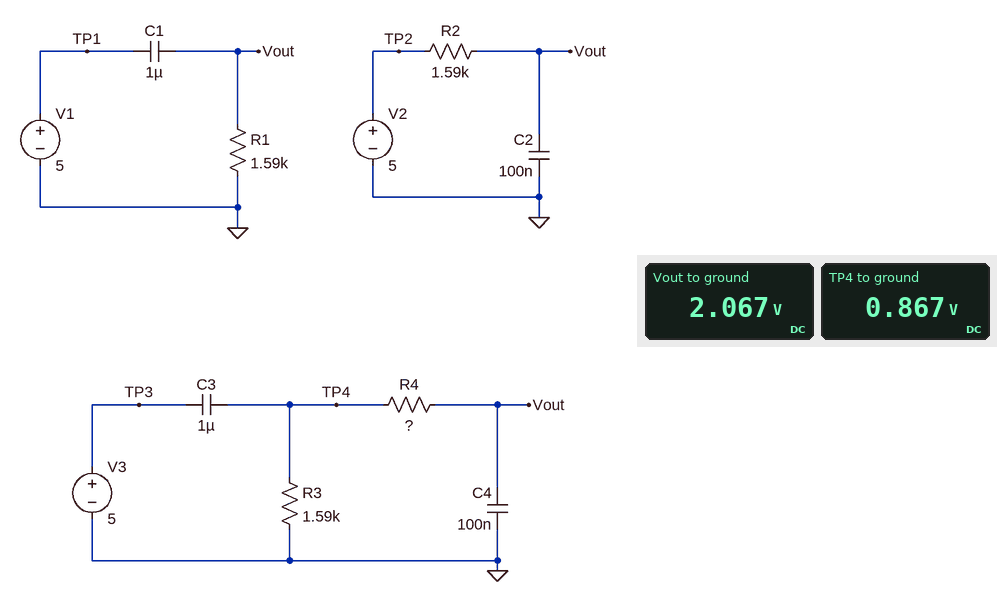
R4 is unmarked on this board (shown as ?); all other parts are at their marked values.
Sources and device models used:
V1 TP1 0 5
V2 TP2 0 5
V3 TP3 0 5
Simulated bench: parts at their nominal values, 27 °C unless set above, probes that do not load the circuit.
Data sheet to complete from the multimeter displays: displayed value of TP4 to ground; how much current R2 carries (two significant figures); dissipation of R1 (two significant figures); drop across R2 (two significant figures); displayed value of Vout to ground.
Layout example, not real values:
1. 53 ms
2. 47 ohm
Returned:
1. 0.867 V
2. 1.8 mA
3. 2.7 mW
4. 2.9 V
5. 2.067 V
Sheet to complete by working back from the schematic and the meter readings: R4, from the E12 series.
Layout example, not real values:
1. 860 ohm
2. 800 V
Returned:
1. 2.2 kΩ
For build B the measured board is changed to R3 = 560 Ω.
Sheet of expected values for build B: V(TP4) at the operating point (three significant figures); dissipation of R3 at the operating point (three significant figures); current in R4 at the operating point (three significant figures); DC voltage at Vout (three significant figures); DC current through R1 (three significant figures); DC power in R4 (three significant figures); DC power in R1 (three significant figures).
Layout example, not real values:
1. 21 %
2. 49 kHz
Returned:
1. 394 mV
2. 277 µW
3. 703 µA
4. 1.94 V
5. 1.22 mA
6. 1.09 mW
7. 2.37 mW
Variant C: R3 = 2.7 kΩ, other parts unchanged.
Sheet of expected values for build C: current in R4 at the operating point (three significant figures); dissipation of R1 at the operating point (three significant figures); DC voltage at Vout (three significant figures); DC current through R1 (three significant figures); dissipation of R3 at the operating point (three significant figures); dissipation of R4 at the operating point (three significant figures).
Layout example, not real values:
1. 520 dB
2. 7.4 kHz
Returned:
1. 439 µA
2. 2.91 mW
3. 2.15 V
4. 1.35 mA
5. 520 µW
6. 424 µW
